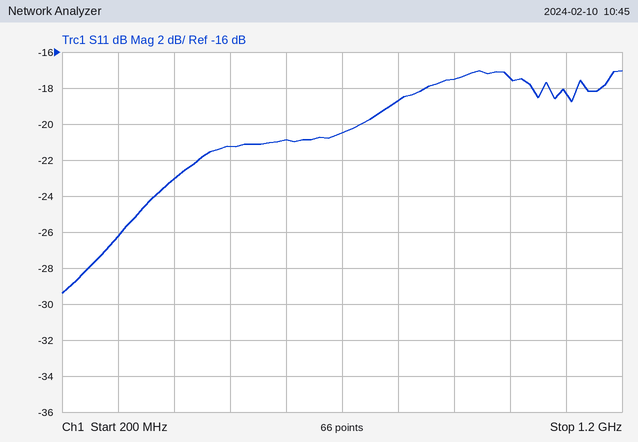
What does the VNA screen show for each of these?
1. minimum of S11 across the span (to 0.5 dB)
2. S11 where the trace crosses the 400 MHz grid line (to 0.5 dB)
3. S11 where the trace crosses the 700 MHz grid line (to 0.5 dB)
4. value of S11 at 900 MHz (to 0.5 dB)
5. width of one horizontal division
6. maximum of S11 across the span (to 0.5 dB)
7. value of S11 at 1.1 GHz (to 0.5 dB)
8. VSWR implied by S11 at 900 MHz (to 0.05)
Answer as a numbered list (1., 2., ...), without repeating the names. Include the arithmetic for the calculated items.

1. -29.5 dB
2. -23.0 dB
3. -20.5 dB
4. -17.5 dB
5. 100 MHz
6. -17.0 dB
7. -18.5 dB
8. |Γ| = 10^(-17.5/20) = 0.1334; VSWR = (1 + 0.1334)/(1 − 0.1334) ≈ 1.31, so 1.30 to the nearest 0.05
